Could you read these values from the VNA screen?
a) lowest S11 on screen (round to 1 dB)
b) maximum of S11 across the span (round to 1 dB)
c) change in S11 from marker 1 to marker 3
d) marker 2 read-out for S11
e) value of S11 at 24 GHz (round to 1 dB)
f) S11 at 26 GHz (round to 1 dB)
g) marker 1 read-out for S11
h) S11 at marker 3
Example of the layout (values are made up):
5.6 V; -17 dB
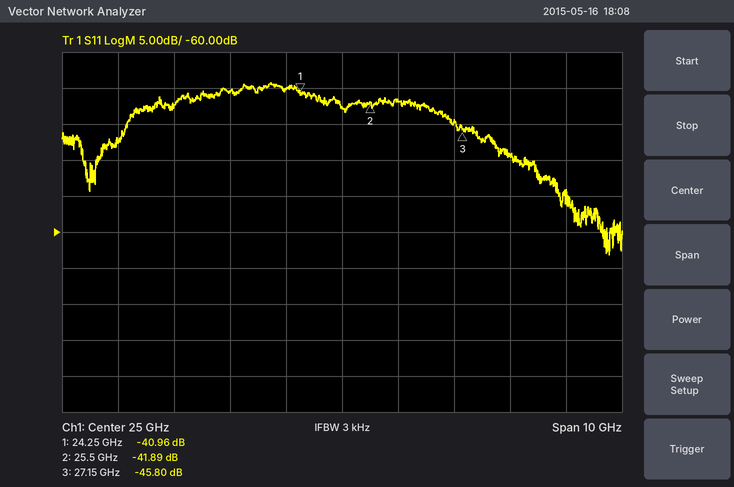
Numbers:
-63 dB; -39 dB; -4.84 dB; -41.89 dB; -40 dB; -42 dB; -40.96 dB; -45.80 dB
